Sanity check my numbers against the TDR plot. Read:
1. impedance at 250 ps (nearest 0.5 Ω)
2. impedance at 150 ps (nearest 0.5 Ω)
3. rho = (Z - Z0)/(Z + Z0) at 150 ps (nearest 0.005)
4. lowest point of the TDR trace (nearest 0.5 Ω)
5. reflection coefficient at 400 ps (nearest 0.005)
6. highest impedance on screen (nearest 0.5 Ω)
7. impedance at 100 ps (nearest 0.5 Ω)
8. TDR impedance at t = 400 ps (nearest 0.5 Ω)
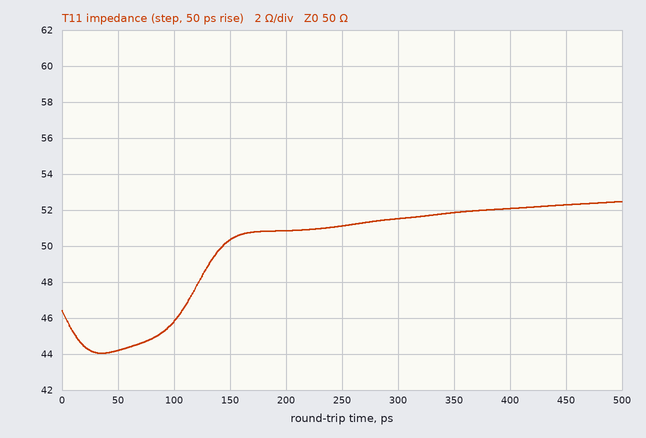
51.0 Ω
50.5 Ω
+0.005
44.0 Ω
+0.020
52.5 Ω
46.0 Ω
52.0 Ω
